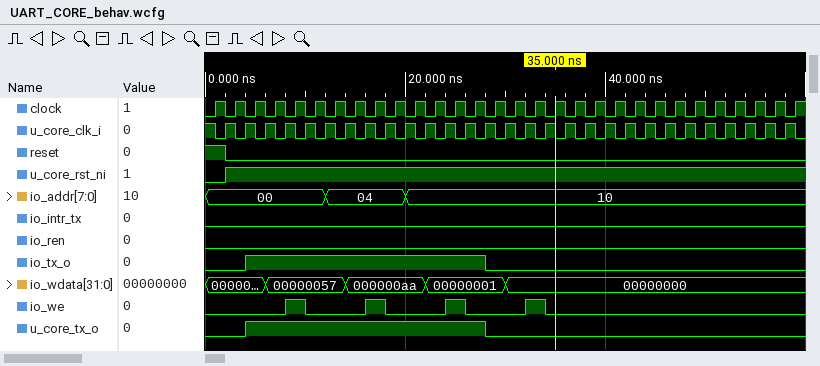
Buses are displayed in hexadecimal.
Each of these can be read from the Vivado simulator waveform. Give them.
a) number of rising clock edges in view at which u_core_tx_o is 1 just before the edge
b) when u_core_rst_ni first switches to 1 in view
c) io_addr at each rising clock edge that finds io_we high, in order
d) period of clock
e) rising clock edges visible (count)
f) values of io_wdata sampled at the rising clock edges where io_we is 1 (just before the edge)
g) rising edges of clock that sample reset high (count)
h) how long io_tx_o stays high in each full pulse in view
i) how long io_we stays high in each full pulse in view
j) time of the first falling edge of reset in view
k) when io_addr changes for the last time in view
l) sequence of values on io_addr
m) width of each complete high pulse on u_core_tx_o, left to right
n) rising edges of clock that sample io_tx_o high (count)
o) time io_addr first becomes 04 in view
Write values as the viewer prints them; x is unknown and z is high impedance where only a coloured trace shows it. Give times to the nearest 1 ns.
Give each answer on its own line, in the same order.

12
2 ns
00, 04, 10, 10
2 ns
30
00000057, 000000aa, 00000001, 00000000
1
24 ns
2 ns, 2 ns, 2 ns, 2 ns
2 ns
20 ns
00, 04, 10
24 ns
12
12 ns
